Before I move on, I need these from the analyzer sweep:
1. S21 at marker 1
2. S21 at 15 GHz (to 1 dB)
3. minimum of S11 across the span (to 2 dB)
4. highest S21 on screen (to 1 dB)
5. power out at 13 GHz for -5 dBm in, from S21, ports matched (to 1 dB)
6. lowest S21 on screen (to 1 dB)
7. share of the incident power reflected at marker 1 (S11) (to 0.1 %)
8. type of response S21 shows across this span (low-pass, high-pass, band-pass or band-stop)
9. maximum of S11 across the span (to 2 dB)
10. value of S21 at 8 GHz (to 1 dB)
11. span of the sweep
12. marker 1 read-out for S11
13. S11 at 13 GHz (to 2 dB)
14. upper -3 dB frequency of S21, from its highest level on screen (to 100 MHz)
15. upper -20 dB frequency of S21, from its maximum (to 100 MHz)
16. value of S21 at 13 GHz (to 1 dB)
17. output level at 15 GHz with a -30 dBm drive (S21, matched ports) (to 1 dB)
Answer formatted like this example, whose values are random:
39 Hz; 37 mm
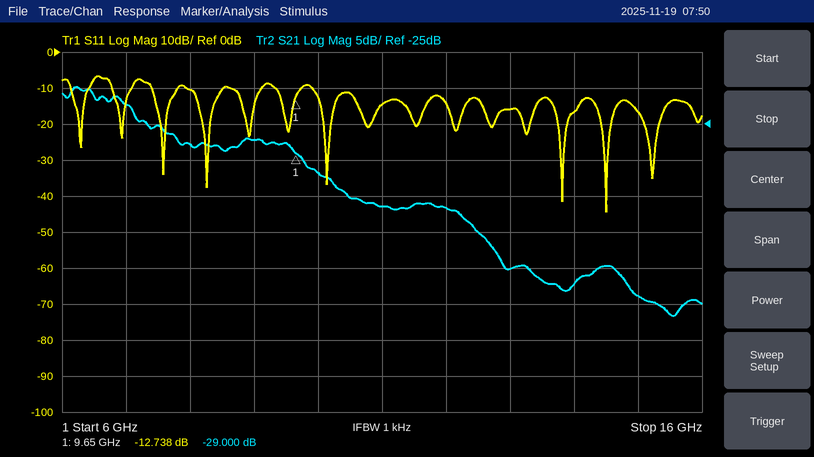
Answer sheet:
-29.000 dB; -49 dB; -44 dB; -20 dB; -50 dBm; -52 dB; 5.3 %; low-pass; -6 dB; -28 dB; 10 GHz; -12.738 dB; -16 dB; 7.1 GHz; 12.5 GHz; -45 dB; -79 dBm
